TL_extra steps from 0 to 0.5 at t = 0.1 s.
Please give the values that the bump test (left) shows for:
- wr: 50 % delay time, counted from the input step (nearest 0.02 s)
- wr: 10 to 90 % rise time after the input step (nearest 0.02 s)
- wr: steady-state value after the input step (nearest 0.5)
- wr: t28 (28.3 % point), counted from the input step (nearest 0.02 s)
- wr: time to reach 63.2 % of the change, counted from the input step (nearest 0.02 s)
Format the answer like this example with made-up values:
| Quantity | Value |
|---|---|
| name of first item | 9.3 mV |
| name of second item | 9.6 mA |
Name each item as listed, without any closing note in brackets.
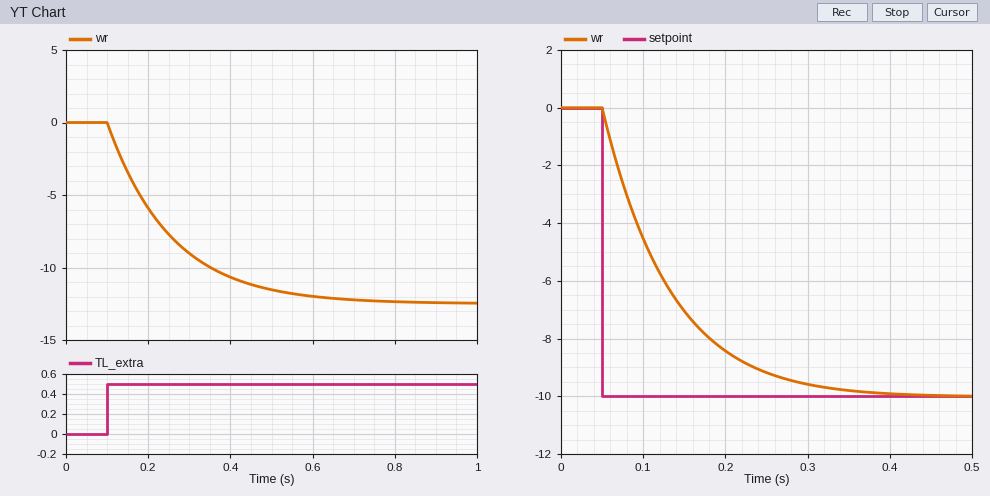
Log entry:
| Quantity | Value |
|---|---|
| wr: 50 % delay time, counted from the input step | 0.10 s |
| wr: 10 to 90 % rise time after the input step | 0.34 s |
| wr: steady-state value after the input step | -12.5 |
| wr: t28 (28.3 % point), counted from the input step | 0.06 s |
| wr: time to reach 63.2 % of the change, counted from the input step | 0.16 s |
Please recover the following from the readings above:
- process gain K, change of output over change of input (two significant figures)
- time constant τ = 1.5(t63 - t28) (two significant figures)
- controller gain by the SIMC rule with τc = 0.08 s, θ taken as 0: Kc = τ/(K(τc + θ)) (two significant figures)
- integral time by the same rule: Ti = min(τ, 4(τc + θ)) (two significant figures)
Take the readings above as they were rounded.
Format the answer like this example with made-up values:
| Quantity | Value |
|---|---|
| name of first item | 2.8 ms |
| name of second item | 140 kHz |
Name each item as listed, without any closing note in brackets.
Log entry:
| Quantity | Value |
|---|---|
| process gain K, change of output over change of input | -25 |
| time constant τ = 1.5(t63 - t28) | 0.15 s |
| controller gain by the SIMC rule with τc = 0.08 s, θ taken as 0: Kc = τ/(K(τc + θ)) | -0.075 |
| integral time by the same rule: Ti = min(τ, 4(τc + θ)) | 0.15 s |
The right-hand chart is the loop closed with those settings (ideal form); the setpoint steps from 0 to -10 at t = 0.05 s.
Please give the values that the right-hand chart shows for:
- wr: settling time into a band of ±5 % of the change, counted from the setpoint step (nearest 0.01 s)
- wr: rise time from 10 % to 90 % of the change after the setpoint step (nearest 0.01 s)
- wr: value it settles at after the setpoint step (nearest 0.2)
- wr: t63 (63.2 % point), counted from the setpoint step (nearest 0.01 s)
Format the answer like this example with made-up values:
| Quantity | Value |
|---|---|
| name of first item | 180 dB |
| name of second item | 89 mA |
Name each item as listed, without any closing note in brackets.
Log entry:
| Quantity | Value |
|---|---|
| wr: settling time into a band of ±5 % of the change, counted from the setpoint step | 0.24 s |
| wr: rise time from 10 % to 90 % of the change after the setpoint step | 0.18 s |
| wr: value it settles at after the setpoint step | -10.0 |
| wr: t63 (63.2 % point), counted from the setpoint step | 0.08 s |
